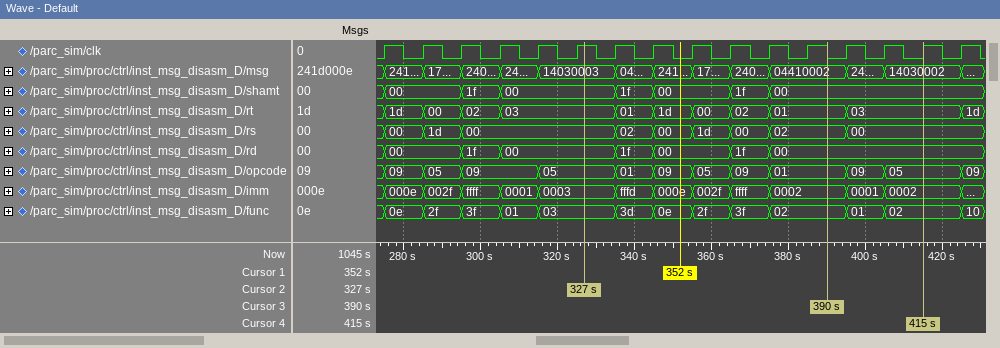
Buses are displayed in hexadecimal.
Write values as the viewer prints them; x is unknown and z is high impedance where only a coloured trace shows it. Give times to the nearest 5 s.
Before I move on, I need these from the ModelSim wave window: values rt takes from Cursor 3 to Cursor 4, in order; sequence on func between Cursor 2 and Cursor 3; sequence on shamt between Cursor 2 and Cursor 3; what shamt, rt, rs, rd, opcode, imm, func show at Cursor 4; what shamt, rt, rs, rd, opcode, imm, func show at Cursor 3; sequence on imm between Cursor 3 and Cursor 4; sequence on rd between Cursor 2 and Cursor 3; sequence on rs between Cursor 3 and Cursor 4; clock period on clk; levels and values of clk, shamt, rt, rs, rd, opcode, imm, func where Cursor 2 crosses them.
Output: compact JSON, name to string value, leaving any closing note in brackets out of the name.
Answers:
{"values rt takes from Cursor 3 to Cursor 4, in order": "01, 03", "sequence on func between Cursor 2 and Cursor 3": "03, 3d, 0e, 2f, 3f, 02", "sequence on shamt between Cursor 2 and Cursor 3": "00, 1f, 00, 1f, 00", "what shamt, rt, rs, rd, opcode, imm, func show at Cursor 4": "shamt=00, rt=03, rs=00, rd=00, opcode=05, imm=0002, func=02", "what shamt, rt, rs, rd, opcode, imm, func show at Cursor 3": "shamt=00, rt=01, rs=02, rd=00, opcode=01, imm=0002, func=02", "sequence on imm between Cursor 3 and Cursor 4": "0002, 0001, 0002", "sequence on rd between Cursor 2 and Cursor 3": "00, 1f, 00, 1f, 00", "sequence on rs between Cursor 3 and Cursor 4": "02, 00", "clock period on clk": "10 s", "levels and values of clk, shamt, rt, rs, rd, opcode, imm, func where Cursor 2 crosses them": "clk=1, shamt=00, rt=03, rs=00, rd=00, opcode=05, imm=0003, func=03"}
